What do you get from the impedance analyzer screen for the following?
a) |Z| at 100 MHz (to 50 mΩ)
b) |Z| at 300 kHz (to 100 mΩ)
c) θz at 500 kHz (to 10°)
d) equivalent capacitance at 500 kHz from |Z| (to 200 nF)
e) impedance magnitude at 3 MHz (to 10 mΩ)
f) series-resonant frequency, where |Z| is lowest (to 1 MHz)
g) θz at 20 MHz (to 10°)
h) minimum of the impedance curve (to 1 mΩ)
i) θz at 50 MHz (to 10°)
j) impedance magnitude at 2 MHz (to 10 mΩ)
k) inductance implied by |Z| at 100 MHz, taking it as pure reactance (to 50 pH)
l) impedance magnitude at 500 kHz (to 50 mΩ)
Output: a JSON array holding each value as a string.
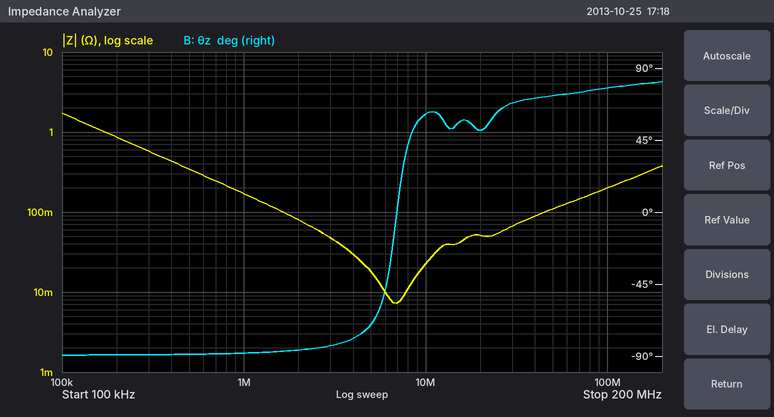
["200 mΩ", "600 mΩ", "-90°", "1.0 µF", "50 mΩ", "7 MHz", "50°", "7 mΩ", "70°", "80 mΩ", "300 pH", "350 mΩ"]
